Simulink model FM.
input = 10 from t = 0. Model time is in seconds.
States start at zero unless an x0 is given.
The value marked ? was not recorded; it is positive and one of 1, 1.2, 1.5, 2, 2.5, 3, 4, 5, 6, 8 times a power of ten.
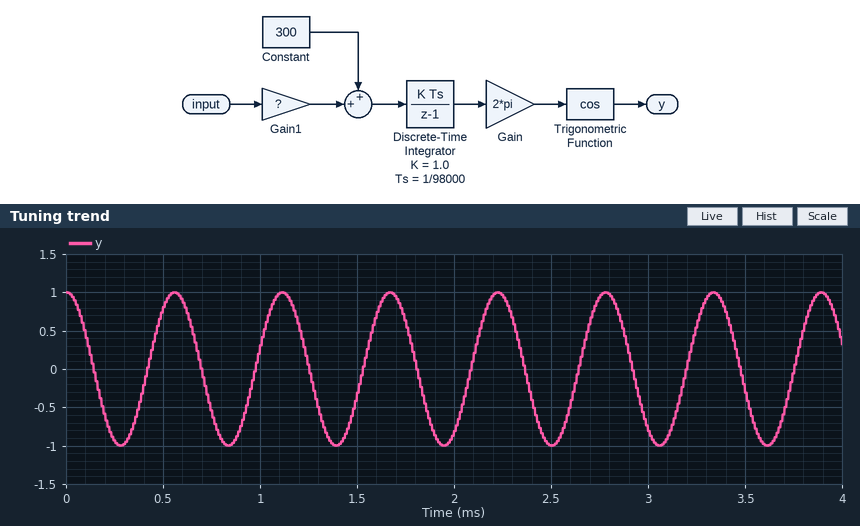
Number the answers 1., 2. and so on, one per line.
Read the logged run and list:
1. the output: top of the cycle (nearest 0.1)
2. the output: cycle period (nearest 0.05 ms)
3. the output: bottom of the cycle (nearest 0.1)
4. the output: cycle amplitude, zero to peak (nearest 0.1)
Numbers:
1. 1.0
2. 0.55 ms
3. -1.0
4. 1.0
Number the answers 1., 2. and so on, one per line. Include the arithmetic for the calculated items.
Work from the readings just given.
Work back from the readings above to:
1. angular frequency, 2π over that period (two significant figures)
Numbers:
1. 2π / 0.55 = 11 rad/ms
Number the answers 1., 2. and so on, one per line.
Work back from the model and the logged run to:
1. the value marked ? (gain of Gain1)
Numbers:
1. 150
